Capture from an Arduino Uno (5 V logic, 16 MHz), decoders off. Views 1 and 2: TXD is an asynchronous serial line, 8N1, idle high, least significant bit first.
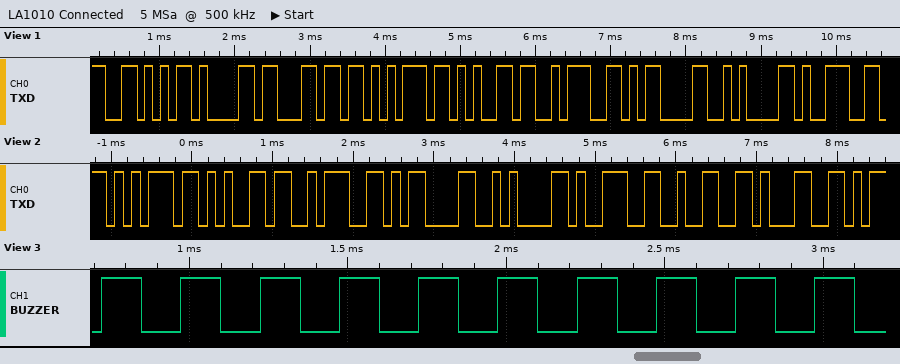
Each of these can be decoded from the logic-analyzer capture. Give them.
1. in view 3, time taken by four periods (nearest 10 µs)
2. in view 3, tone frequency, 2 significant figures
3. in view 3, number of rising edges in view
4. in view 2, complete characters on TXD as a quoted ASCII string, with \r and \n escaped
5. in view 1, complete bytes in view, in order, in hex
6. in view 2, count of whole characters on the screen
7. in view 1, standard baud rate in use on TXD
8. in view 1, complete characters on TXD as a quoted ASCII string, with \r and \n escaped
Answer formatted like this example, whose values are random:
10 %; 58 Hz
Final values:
1000 µs; 4.0 kHz; 10; "ue:\r\n921"; 56 61 6C 75 65 3A 0D 0A 39; 8; 9600 baud; "Value:\r\n9"
